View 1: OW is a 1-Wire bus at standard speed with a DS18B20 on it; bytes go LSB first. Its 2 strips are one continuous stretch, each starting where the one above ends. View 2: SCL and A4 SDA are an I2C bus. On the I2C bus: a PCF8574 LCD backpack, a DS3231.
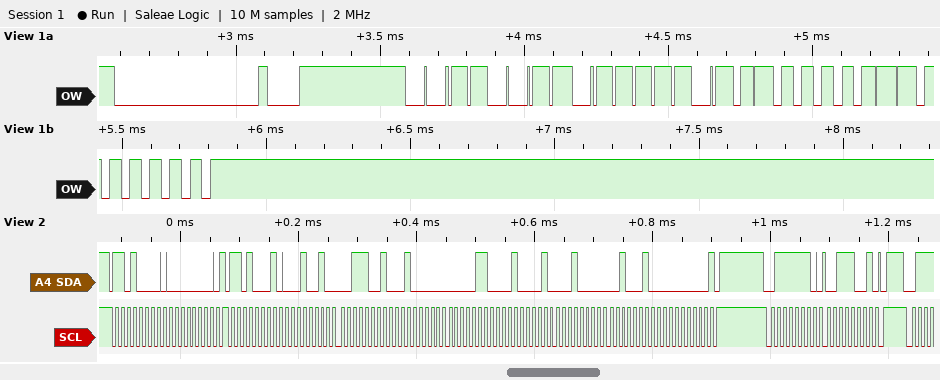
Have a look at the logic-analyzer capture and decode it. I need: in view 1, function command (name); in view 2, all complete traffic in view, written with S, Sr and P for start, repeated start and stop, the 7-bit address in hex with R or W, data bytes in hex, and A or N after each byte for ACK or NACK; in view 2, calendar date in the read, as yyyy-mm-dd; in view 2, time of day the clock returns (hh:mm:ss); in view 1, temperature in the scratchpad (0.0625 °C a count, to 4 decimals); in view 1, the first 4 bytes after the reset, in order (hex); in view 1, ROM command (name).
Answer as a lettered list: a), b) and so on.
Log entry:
a) Read Scratchpad
b) S 68W A 00 A Sr 68R A 12 A 39 A 20 A 06 A 21 A 10 A 22 A 00 N P S 3FW A 39 A P
c) 2022-10-21
d) 20:39:12
e) 24.1250 °C
f) CC BE 82 01
g) Skip ROM
